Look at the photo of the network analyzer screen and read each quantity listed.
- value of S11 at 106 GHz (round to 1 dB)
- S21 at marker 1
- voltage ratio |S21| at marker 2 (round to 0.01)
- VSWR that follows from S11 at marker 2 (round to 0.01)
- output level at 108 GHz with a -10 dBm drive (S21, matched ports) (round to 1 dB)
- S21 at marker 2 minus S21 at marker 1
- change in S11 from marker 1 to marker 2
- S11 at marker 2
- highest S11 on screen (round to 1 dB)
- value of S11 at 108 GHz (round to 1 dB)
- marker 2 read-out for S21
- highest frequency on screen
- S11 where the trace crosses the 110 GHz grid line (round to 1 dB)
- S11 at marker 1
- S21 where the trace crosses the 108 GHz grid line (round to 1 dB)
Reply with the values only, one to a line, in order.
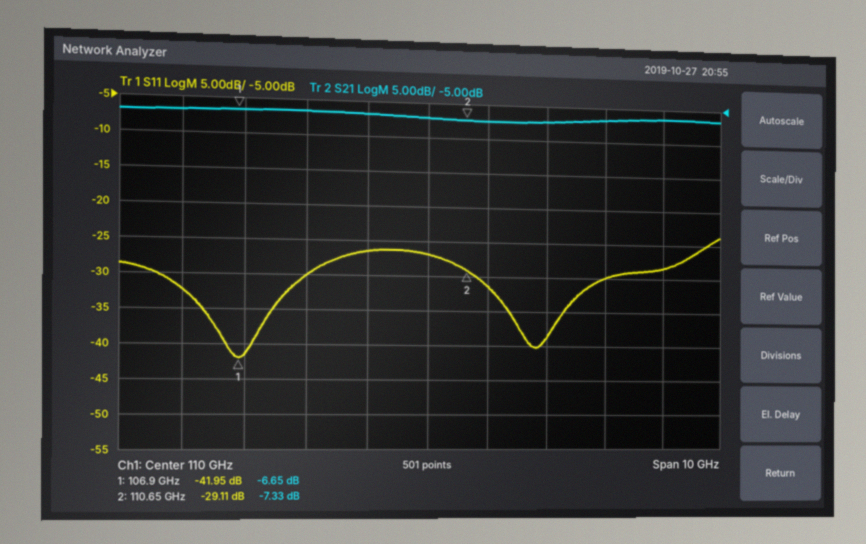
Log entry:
-32 dB
-6.65 dB
0.43
1.07
-17 dBm
-0.68 dB
12.84 dB
-29.11 dB
-24 dB
-30 dB
-7.33 dB
115 GHz
-27 dB
-41.95 dB
-7 dB
